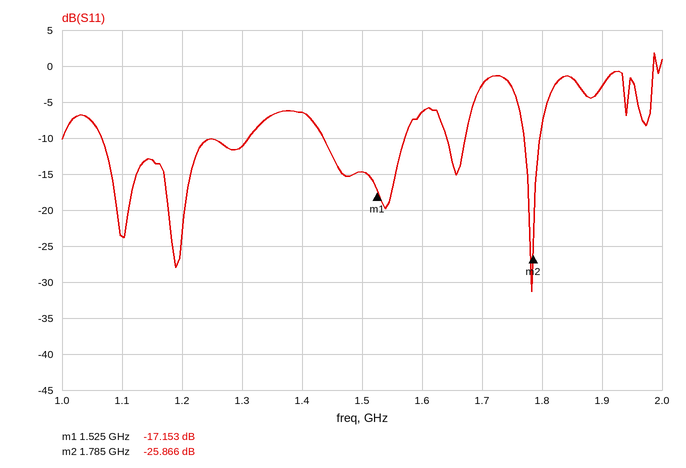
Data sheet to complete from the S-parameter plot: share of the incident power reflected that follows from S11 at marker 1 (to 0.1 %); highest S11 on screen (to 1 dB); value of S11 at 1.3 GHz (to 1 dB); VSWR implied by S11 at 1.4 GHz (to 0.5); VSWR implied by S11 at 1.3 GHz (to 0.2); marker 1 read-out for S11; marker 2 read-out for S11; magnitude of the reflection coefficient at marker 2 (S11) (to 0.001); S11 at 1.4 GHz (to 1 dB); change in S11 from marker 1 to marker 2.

1.9 %
2 dB
-11 dB
3.0
1.8
-17.153 dB
-25.866 dB
0.051
-6 dB
-8.713 dB
